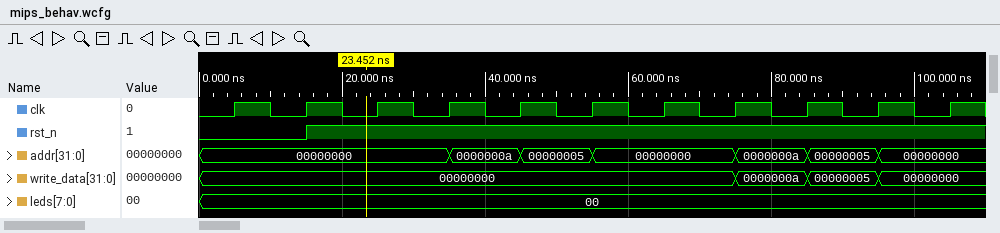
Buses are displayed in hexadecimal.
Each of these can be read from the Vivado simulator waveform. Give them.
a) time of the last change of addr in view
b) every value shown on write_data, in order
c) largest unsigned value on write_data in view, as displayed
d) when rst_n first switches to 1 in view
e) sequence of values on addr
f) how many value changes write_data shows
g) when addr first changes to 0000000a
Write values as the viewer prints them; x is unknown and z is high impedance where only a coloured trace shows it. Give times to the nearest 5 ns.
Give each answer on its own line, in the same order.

95 ns
00000000, 0000000a, 00000005, 00000000
0000000a
15 ns
00000000, 0000000a, 00000005, 00000000, 0000000a, 00000005, 00000000
3
35 ns
